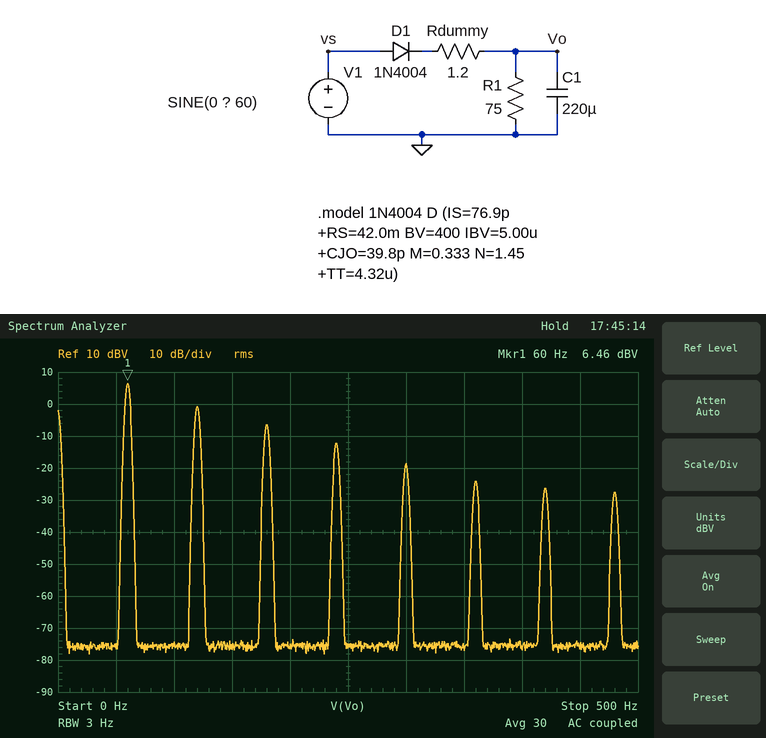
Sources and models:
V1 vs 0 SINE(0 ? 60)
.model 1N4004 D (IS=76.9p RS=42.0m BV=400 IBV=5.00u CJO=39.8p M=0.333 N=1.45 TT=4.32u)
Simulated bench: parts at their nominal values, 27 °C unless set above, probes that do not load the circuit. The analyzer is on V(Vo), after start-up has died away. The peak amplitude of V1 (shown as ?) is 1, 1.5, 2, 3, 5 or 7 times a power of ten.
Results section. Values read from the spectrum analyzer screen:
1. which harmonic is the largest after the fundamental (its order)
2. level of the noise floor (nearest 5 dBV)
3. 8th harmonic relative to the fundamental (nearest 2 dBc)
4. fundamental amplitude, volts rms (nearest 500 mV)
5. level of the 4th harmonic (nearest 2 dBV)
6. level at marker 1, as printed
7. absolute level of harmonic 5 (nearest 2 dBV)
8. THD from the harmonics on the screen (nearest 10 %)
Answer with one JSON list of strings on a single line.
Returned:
["2", "-75 dBV", "-34 dBc", "2.0 V", "-12 dBV", "6.46 dBV", "-18 dBV", "50 %"]
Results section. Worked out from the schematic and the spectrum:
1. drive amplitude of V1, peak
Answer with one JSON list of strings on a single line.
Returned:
["15 V"]
